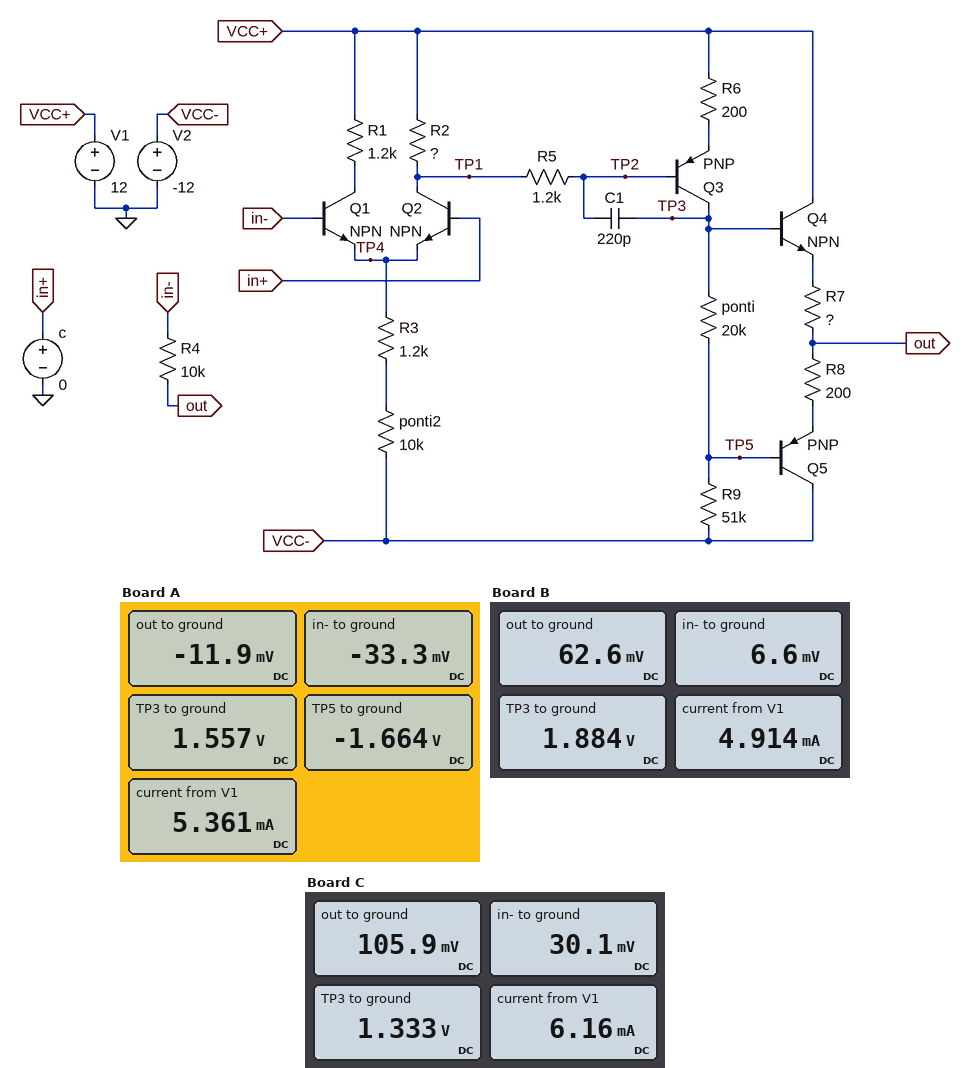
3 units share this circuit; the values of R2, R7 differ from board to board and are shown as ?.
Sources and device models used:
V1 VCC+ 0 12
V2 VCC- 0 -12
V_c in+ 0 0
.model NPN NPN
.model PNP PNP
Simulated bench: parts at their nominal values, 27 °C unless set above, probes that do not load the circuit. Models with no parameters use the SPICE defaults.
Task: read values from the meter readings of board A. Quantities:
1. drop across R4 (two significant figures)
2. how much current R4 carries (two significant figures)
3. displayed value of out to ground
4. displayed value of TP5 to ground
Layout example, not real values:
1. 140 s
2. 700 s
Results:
1. 21 mV
2. 2.1 µA
3. -11.9 mV
4. -1.664 V
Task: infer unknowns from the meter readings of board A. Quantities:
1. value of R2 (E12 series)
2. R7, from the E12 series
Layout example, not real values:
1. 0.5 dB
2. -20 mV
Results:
1. 1 kΩ
2. 180 Ω
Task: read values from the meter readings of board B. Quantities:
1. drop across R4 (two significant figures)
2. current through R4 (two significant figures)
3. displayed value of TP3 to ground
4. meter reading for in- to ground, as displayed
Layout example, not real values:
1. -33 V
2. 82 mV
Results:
1. 56 mV
2. 5.6 µA
3. 1.884 V
4. 6.6 mV
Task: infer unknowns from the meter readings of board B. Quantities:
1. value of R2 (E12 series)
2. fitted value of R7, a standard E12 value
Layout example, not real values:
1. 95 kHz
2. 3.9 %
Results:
1. 1.8 kΩ
2. 270 Ω
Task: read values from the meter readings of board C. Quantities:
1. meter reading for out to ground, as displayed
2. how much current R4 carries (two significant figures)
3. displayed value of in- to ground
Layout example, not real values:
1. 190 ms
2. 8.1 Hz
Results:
1. 105.9 mV
2. 7.6 µA
3. 30.1 mV
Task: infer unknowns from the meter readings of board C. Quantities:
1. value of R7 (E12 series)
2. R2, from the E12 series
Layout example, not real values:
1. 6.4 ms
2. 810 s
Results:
1. 82 Ω
2. 3.3 kΩ
